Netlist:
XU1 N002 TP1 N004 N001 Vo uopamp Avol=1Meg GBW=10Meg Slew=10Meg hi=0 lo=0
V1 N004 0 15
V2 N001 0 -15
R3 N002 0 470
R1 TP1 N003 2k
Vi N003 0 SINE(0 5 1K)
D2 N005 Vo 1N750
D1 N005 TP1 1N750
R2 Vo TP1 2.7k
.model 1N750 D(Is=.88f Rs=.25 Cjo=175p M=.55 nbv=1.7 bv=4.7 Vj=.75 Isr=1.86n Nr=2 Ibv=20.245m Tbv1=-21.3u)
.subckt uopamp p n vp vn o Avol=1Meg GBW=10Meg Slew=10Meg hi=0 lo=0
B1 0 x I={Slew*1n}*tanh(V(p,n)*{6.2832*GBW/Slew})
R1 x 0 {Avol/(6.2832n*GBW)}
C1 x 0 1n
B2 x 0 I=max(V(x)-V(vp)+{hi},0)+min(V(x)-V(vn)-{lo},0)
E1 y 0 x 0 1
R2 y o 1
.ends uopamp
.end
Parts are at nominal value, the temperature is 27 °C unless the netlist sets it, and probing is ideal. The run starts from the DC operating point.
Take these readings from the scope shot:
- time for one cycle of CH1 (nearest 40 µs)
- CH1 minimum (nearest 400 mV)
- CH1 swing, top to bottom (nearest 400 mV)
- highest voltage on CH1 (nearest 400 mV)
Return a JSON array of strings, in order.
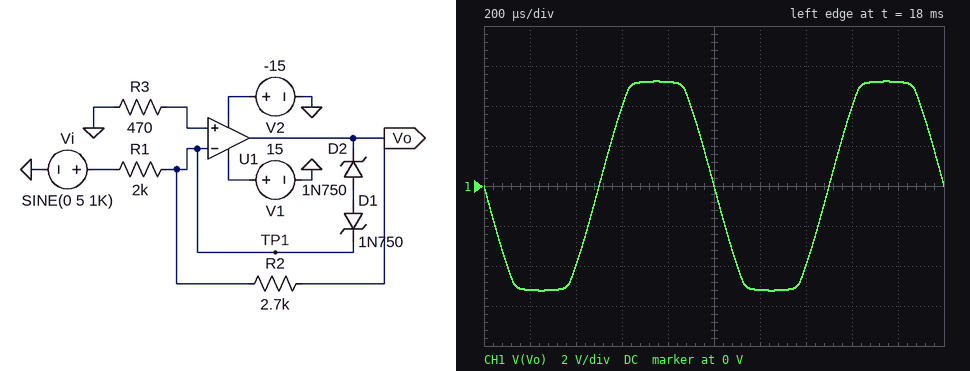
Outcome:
["1.00 ms", "-5.2 V", "10.4 V", "5.2 V"]
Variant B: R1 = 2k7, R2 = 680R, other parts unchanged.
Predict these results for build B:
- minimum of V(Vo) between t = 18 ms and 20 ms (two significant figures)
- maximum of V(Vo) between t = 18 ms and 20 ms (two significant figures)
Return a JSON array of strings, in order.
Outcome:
["-1.3 V", "1.3 V"]
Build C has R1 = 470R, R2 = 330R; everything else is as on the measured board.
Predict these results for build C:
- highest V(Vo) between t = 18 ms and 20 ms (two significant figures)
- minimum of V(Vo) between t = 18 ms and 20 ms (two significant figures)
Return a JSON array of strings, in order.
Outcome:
["3.5 V", "-3.5 V"]
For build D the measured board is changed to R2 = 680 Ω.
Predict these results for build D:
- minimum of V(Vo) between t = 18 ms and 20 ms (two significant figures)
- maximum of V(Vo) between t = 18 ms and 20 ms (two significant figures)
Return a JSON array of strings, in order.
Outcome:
["-1.7 V", "1.7 V"]
